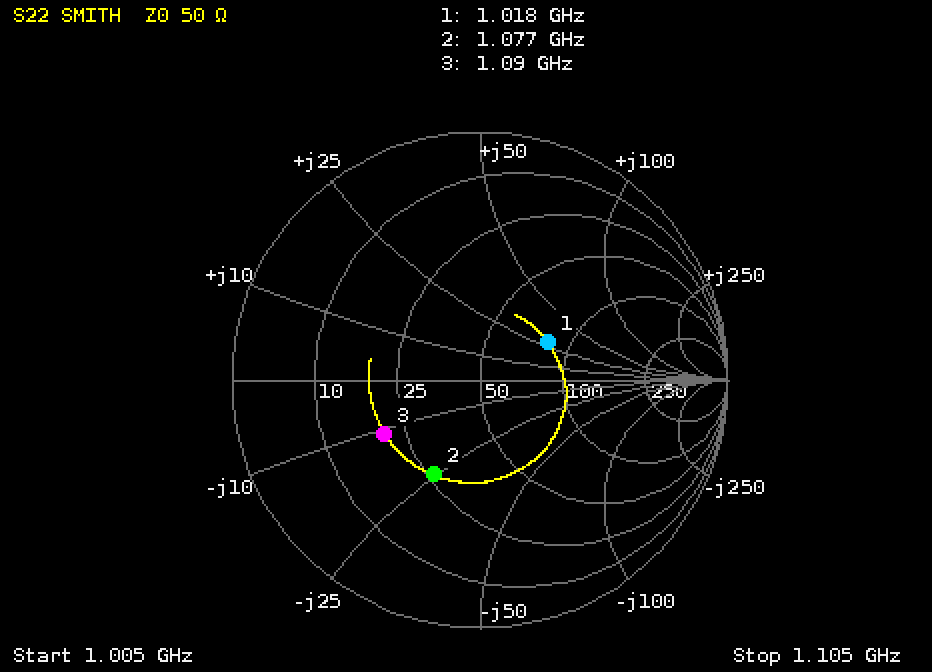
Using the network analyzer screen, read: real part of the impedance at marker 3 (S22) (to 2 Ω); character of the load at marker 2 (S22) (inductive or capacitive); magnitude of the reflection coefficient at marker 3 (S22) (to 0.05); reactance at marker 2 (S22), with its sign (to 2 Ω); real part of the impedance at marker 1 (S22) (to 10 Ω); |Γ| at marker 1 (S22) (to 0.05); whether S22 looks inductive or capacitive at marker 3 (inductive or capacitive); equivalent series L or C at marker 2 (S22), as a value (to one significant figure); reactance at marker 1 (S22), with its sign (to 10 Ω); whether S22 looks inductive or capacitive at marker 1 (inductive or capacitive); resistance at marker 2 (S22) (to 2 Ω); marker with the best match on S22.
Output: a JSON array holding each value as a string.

["20 Ω", "capacitive", "0.45", "-24 Ω", "80 Ω", "0.30", "capacitive", "6 pF", "+30 Ω", "inductive", "26 Ω", "marker 1"]
